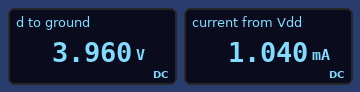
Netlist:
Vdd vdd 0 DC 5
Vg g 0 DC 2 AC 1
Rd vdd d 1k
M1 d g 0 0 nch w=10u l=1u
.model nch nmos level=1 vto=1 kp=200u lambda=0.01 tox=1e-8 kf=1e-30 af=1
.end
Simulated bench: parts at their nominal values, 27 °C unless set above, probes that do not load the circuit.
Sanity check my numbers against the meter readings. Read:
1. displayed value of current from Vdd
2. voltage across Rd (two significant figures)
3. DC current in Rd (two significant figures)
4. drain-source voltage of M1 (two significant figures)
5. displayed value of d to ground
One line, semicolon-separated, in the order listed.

1.040 mA; 1.0 V; 1.0 mA; 4.0 V; 3.960 V
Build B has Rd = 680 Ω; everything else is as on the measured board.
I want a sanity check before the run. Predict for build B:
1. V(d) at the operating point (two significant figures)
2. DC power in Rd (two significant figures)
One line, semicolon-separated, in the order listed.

4.3 V; 740 µW
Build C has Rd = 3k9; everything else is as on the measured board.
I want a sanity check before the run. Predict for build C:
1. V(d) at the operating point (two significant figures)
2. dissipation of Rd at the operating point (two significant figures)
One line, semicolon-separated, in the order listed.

1.1 V; 4.0 mW
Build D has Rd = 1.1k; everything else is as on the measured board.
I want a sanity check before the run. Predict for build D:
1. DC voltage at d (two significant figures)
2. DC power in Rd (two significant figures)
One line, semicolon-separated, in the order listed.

3.9 V; 1.2 mW
